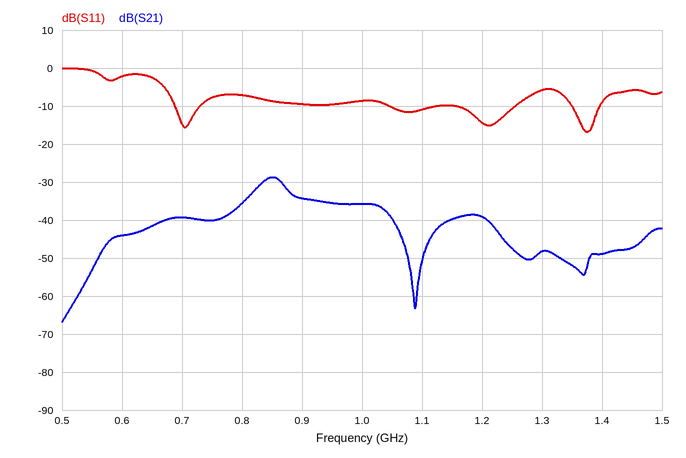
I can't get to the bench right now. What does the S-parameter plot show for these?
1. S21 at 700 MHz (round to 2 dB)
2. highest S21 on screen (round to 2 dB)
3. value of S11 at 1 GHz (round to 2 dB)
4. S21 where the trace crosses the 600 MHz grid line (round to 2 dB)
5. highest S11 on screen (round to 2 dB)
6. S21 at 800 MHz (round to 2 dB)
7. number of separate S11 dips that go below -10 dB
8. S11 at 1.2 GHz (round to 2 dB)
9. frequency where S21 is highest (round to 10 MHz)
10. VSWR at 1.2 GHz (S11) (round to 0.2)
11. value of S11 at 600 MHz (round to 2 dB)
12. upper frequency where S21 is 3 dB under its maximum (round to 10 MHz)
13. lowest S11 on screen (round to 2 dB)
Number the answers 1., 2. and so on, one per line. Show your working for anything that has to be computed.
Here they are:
1. -40 dB
2. -28 dB
3. -8 dB
4. -44 dB
5. 0 dB
6. -36 dB
7. 3
8. -14 dB
9. 850 MHz
10. |Γ| = 10^(-14/20) = 0.1995; VSWR = (1 + 0.1995)/(1 − 0.1995) ≈ 1.50, so 1.4 to the nearest 0.2
11. -2 dB
12. 870 MHz
13. -16 dB
